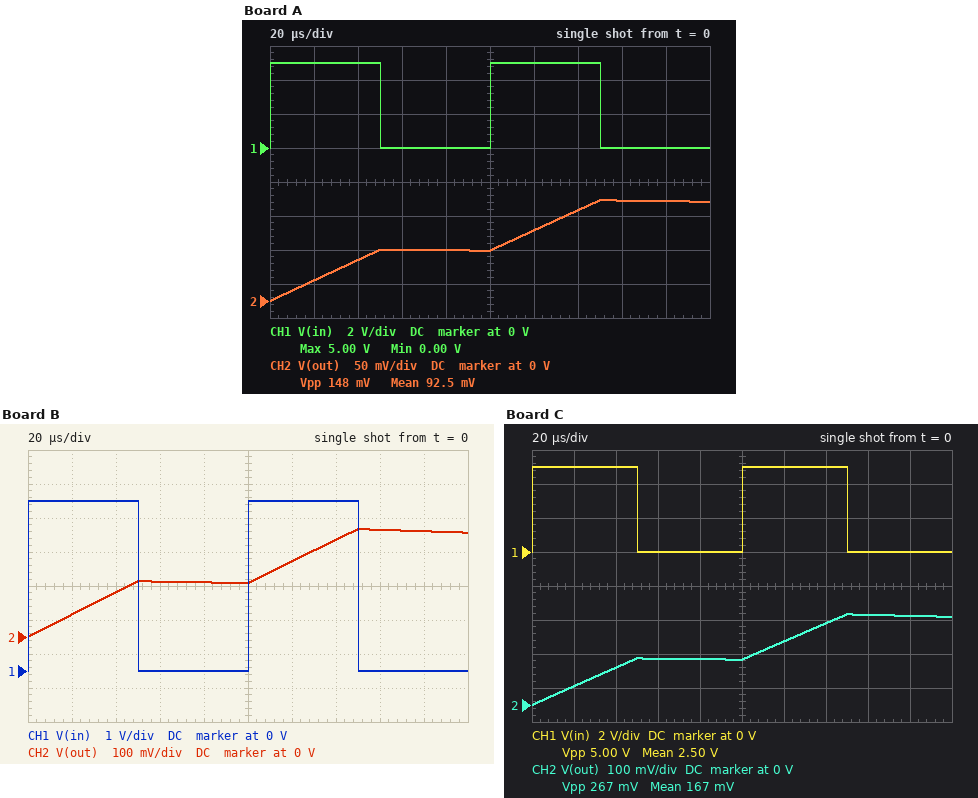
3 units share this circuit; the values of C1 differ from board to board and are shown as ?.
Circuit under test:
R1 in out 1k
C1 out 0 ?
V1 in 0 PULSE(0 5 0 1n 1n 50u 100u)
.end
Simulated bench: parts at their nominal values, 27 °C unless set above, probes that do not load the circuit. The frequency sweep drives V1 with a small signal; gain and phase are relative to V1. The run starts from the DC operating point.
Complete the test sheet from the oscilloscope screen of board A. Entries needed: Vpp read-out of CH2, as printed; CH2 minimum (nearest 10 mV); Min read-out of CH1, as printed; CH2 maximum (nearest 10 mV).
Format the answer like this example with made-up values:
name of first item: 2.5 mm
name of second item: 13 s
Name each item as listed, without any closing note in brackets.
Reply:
Vpp read-out of CH2, as printed: 148 mV
CH2 minimum: 0 V
Min read-out of CH1, as printed: 0.00 V
CH2 maximum: 150 mV
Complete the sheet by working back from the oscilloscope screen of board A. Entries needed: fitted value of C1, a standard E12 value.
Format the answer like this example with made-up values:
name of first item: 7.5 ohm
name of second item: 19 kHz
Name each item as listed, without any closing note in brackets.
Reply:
fitted value of C1, a standard E12 value: 3.3 µF
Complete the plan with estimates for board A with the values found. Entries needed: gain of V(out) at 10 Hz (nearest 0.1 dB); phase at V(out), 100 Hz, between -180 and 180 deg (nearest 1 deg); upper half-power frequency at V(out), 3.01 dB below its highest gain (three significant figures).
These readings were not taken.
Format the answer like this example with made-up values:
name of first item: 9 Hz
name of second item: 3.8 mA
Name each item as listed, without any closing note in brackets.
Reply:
gain of V(out) at 10 Hz: -0.2 dB
phase at V(out), 100 Hz, between -180 and 180 deg: -64 deg
upper half-power frequency at V(out), 3.01 dB below its highest gain: 48.2 Hz
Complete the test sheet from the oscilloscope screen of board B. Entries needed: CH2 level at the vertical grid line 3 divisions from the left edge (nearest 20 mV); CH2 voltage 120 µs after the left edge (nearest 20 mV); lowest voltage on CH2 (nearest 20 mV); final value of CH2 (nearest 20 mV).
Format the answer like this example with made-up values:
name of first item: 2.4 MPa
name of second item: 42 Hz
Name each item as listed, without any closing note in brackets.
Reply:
CH2 level at the vertical grid line 3 divisions from the left edge: 160 mV
CH2 voltage 120 µs after the left edge: 220 mV
lowest voltage on CH2: 0 V
final value of CH2: 300 mV
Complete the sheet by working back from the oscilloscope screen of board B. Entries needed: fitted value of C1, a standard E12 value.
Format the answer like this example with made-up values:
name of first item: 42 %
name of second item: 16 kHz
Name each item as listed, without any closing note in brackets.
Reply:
fitted value of C1, a standard E12 value: 1.5 µF
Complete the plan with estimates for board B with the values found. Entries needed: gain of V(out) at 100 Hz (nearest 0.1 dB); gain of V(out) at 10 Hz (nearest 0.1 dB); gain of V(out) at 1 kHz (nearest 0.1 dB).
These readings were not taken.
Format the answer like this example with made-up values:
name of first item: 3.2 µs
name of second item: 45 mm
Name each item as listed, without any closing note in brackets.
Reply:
gain of V(out) at 100 Hz: -2.8 dB
gain of V(out) at 10 Hz: 0 dB
gain of V(out) at 1 kHz: -19.5 dB
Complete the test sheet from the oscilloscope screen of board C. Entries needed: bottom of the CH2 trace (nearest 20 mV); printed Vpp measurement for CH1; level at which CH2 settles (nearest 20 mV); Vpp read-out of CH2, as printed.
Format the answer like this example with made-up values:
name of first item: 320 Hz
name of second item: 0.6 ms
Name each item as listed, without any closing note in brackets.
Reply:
bottom of the CH2 trace: 0 V
printed Vpp measurement for CH1: 5.00 V
level at which CH2 settles: 260 mV
Vpp read-out of CH2, as printed: 267 mV
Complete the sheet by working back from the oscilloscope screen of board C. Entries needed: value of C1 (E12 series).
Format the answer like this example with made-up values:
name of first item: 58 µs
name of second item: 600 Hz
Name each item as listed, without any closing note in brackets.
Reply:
value of C1: 1.8 µF
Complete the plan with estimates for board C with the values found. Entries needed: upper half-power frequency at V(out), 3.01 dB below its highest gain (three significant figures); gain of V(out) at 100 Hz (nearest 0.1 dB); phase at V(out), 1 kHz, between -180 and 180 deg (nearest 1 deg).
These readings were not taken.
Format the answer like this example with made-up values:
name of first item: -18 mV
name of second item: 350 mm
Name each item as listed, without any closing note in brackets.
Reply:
upper half-power frequency at V(out), 3.01 dB below its highest gain: 88.4 Hz
gain of V(out) at 100 Hz: -3.6 dB
phase at V(out), 1 kHz, between -180 and 180 deg: -85 deg
